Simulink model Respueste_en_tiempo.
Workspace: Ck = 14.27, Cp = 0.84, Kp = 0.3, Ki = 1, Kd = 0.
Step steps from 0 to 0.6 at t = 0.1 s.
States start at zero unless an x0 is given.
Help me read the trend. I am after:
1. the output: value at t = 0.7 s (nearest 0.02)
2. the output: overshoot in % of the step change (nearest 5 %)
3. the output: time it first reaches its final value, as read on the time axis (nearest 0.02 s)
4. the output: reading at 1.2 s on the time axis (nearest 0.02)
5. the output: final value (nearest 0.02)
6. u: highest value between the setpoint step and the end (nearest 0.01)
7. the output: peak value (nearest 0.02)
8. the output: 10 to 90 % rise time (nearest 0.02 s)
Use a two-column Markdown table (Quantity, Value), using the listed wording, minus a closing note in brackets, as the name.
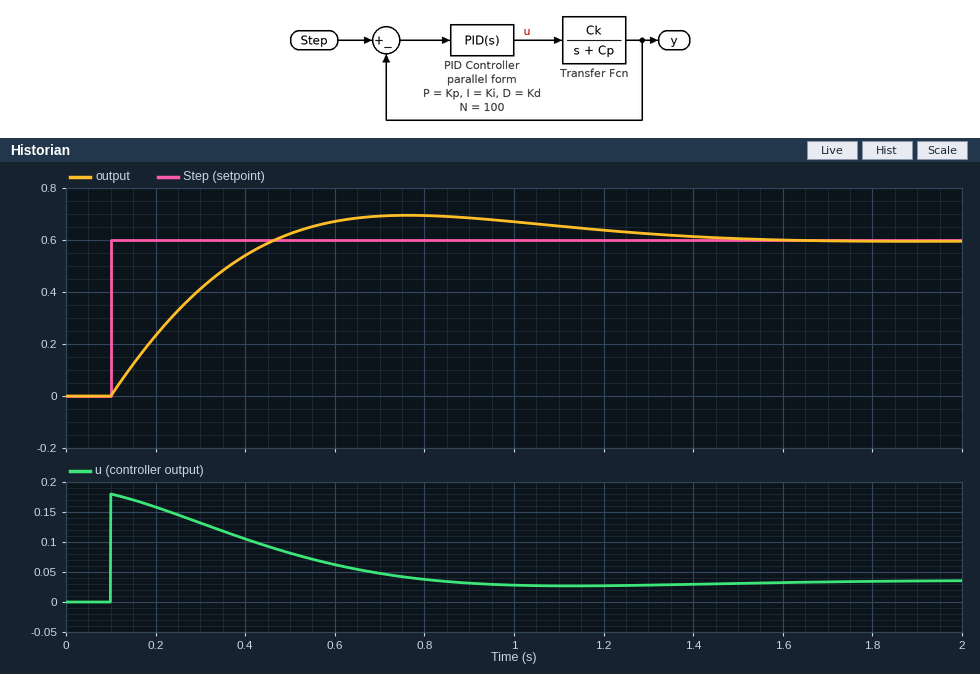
| Quantity | Value |
|---|---|
| the output: value at t = 0.7 s | 0.70 |
| the output: overshoot in % of the step change | 15 % |
| the output: time it first reaches its final value, as read on the time axis | 0.46 s |
| the output: reading at 1.2 s on the time axis | 0.64 |
| the output: final value | 0.60 |
| u: highest value between the setpoint step and the end | 0.18 |
| the output: peak value | 0.70 |
| the output: 10 to 90 % rise time | 0.28 s |
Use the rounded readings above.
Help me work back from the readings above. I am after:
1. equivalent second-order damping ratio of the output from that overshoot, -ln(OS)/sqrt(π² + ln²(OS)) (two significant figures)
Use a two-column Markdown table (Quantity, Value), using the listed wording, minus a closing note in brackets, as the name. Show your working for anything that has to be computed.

| Quantity | Value |
|---|---|
| equivalent second-order damping ratio of the output from that overshoot, -ln(OS)/sqrt(π² + ln²(OS)) | ln(0.15) = -1.897; 1.897 / sqrt(9.870 + 3.599) = 0.52 |
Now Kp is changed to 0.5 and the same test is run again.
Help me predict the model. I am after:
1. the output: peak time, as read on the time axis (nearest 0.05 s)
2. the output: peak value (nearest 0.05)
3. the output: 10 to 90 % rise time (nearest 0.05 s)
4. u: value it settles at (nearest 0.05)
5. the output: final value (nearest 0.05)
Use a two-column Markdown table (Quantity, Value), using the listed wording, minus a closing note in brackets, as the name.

| Quantity | Value |
|---|---|
| the output: peak time, as read on the time axis | 0.70 s |
| the output: peak value | 0.65 |
| the output: 10 to 90 % rise time | 0.25 s |
| u: value it settles at | 0.05 |
| the output: final value | 0.60 |
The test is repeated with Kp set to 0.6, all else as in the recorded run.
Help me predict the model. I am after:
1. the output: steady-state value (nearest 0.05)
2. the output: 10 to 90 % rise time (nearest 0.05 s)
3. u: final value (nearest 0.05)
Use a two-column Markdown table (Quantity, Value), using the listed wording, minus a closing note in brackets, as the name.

| Quantity | Value |
|---|---|
| the output: steady-state value | 0.60 |
| the output: 10 to 90 % rise time | 0.20 s |
| u: final value | 0.05 |
